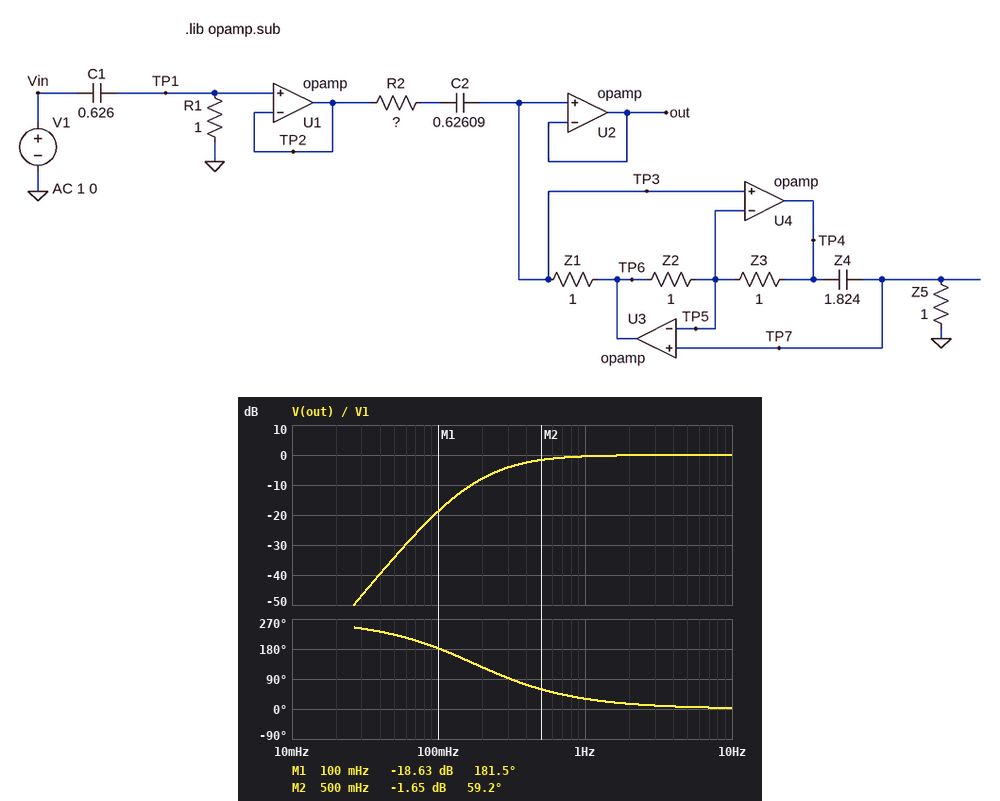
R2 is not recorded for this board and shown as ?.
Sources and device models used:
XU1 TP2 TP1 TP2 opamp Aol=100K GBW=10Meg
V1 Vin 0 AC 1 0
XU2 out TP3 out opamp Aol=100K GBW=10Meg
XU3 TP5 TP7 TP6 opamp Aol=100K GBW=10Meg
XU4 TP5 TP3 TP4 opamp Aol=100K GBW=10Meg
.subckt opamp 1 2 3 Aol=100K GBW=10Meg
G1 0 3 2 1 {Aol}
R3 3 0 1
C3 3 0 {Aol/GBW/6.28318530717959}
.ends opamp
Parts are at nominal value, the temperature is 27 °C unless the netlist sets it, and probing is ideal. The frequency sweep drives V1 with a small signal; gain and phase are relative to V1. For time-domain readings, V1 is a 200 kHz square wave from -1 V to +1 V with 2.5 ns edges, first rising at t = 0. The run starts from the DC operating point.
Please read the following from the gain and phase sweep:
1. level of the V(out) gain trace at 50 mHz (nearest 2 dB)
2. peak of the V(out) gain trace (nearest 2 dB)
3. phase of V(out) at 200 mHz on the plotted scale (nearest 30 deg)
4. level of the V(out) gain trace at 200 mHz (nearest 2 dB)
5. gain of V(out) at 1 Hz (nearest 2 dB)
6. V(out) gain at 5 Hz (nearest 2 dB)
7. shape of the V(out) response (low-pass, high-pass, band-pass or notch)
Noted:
-34 dB
0 dB
120 deg
-8 dB
0 dB
0 dB
high-pass
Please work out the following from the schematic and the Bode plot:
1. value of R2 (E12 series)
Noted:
3.3 Ω
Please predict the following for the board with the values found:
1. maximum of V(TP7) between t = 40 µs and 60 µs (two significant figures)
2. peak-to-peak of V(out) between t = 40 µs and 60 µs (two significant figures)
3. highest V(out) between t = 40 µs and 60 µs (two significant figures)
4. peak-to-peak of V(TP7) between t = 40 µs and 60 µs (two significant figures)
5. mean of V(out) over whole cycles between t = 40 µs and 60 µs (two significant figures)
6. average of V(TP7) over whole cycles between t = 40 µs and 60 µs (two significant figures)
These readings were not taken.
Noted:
2.0 V
2.0 V
2.0 V
2.0 V
1.0 V
1.0 V
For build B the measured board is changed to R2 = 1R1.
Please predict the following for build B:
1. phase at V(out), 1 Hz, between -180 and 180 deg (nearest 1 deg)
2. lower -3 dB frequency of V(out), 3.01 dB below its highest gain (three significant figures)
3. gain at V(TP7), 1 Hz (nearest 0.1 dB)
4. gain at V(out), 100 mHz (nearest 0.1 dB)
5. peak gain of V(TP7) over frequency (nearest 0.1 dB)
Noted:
20 deg
141 mHz
-0.1 dB
-12.5 dB
0 dB
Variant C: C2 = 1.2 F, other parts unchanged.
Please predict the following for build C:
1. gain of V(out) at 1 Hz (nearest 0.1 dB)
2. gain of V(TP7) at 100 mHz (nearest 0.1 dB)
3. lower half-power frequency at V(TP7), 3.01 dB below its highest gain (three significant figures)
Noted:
-0.5 dB
-17.9 dB
389 mHz
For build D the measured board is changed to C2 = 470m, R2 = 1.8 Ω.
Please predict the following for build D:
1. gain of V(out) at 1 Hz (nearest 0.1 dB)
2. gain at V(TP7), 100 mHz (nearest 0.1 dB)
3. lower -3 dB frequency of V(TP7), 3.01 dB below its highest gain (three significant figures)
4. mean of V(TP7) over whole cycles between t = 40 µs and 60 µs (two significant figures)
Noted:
-0.1 dB
-16.7 dB
190 mHz
1.0 V
